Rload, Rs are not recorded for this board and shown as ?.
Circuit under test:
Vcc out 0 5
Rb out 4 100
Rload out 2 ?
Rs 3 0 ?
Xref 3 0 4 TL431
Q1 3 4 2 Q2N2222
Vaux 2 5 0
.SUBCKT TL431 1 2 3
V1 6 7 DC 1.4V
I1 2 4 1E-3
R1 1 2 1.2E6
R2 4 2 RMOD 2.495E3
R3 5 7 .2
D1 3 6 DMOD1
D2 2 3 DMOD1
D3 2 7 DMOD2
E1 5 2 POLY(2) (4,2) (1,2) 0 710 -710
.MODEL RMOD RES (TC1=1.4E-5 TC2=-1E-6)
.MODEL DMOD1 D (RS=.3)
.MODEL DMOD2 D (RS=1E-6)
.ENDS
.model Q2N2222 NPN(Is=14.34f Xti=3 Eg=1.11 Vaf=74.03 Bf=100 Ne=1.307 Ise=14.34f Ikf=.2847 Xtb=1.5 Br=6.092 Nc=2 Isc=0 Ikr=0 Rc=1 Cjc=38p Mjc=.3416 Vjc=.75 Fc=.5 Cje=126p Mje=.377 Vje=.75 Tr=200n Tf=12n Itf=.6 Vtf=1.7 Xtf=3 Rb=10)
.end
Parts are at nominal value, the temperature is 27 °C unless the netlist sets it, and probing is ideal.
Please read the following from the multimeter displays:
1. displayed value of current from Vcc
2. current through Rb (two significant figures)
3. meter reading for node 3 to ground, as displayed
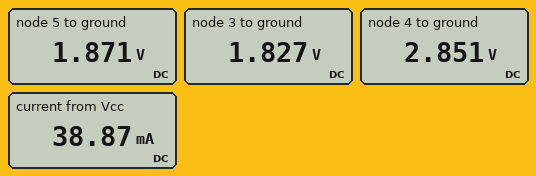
38.87 mA
21 mA
1.827 V
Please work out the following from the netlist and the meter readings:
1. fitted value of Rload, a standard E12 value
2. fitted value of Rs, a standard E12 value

180 Ω
47 Ω
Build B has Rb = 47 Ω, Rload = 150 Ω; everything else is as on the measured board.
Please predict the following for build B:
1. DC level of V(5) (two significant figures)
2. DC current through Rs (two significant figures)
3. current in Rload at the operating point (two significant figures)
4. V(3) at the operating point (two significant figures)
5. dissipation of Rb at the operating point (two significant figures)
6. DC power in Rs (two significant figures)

2.4 V
50 mA
17 mA
2.3 V
49 mW
120 mW
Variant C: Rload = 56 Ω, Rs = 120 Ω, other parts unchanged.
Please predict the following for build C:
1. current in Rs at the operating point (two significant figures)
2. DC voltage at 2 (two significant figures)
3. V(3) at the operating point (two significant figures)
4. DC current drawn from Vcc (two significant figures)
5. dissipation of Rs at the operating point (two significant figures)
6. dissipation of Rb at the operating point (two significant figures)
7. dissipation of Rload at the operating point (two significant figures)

21 mA
4.0 V
2.5 V
35 mA
52 mW
30 mW
18 mW
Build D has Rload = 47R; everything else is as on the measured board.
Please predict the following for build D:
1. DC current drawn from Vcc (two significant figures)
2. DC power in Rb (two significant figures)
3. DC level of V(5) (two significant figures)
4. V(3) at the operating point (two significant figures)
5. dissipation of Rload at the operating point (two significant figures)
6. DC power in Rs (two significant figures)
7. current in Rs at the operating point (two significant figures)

62 mA
27 mW
2.9 V
2.5 V
97 mW
130 mW
53 mA
